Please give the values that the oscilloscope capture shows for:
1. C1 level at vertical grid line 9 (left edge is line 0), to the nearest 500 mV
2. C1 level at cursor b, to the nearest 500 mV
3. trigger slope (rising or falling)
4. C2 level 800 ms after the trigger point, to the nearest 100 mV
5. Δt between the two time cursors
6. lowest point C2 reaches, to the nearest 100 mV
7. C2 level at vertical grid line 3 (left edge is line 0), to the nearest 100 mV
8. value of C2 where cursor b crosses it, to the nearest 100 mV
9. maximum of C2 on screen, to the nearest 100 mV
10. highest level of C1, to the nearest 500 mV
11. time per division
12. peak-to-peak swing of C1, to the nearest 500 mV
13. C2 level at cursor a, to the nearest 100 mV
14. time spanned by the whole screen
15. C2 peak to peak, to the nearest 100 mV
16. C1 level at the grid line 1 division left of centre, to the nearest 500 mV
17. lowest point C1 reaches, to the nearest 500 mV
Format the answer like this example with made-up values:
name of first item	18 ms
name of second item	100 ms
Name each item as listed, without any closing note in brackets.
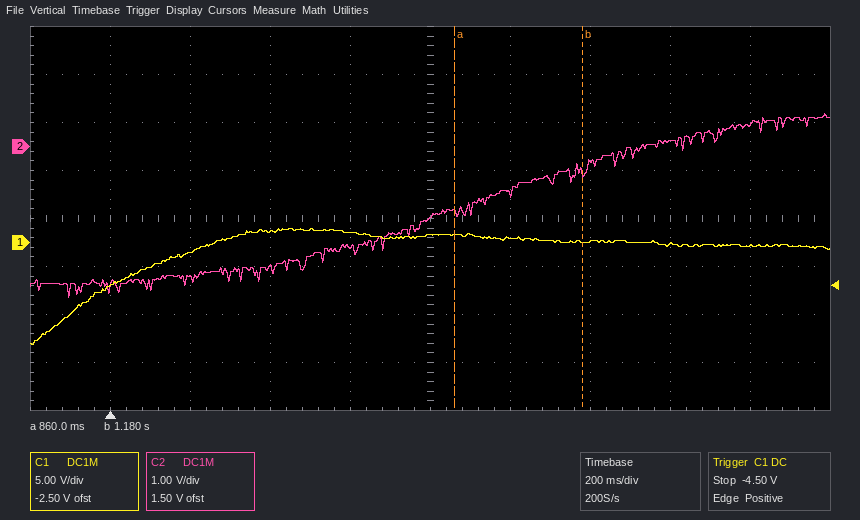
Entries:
C1 level at vertical grid line 9 (left edge is line 0), to the nearest 500 mV	-500 mV
C1 level at cursor b, to the nearest 500 mV	0.0 V
trigger slope	rising
C2 level 800 ms after the trigger point, to the nearest 100 mV	-1.5 V
Δt between the two time cursors	320 ms
lowest point C2 reaches, to the nearest 100 mV	-3.1 V
C2 level at vertical grid line 3 (left edge is line 0), to the nearest 100 mV	-2.6 V
value of C2 where cursor b crosses it, to the nearest 100 mV	-500 mV
maximum of C2 on screen, to the nearest 100 mV	700 mV
highest level of C1, to the nearest 500 mV	1.5 V
time per division	200 ms
peak-to-peak swing of C1, to the nearest 500 mV	12.0 V
C2 level at cursor a, to the nearest 100 mV	-1.4 V
time spanned by the whole screen	2 s
C2 peak to peak, to the nearest 100 mV	3.8 V
C1 level at the grid line 1 division left of centre, to the nearest 500 mV	1.0 V
lowest point C1 reaches, to the nearest 500 mV	-10.5 V
